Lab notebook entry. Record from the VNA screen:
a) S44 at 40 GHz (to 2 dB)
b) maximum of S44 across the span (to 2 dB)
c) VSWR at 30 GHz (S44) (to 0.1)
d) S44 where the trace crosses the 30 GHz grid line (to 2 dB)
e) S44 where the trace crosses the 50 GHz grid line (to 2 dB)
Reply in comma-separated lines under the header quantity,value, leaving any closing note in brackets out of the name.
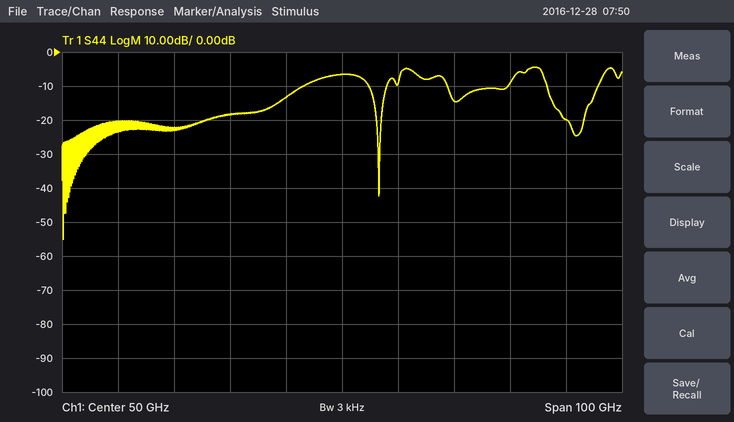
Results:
quantity,value
S44 at 40 GHz,-14 dB
maximum of S44 across the span,-4 dB
VSWR at 30 GHz (S44),1.3
S44 where the trace crosses the 30 GHz grid line,-18 dB
S44 where the trace crosses the 50 GHz grid line,-6 dB
